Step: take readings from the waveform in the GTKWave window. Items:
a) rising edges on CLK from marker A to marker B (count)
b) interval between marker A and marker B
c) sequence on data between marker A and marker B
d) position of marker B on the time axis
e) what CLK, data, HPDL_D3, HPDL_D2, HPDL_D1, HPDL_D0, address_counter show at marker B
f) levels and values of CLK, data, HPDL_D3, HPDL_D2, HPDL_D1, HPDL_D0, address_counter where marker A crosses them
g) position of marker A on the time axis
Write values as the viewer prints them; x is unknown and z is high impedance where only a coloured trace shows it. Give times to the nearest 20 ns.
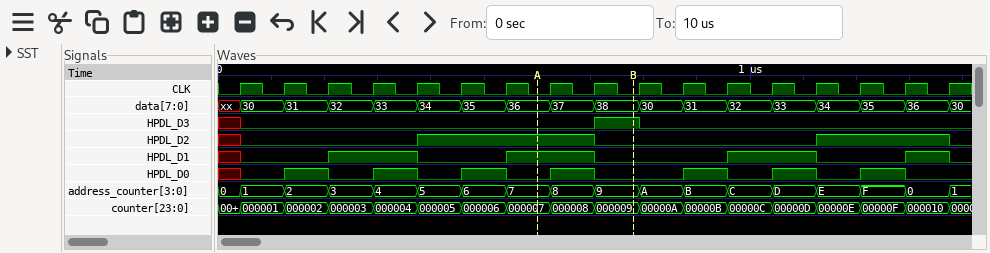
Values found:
2
180 ns
36, 37, 38
780 ns
CLK=0, data=38, HPDL_D3=1, HPDL_D2=0, HPDL_D1=0, HPDL_D0=0, address_counter=9
CLK=0, data=36, HPDL_D3=0, HPDL_D2=1, HPDL_D1=1, HPDL_D0=0, address_counter=7
600 ns
